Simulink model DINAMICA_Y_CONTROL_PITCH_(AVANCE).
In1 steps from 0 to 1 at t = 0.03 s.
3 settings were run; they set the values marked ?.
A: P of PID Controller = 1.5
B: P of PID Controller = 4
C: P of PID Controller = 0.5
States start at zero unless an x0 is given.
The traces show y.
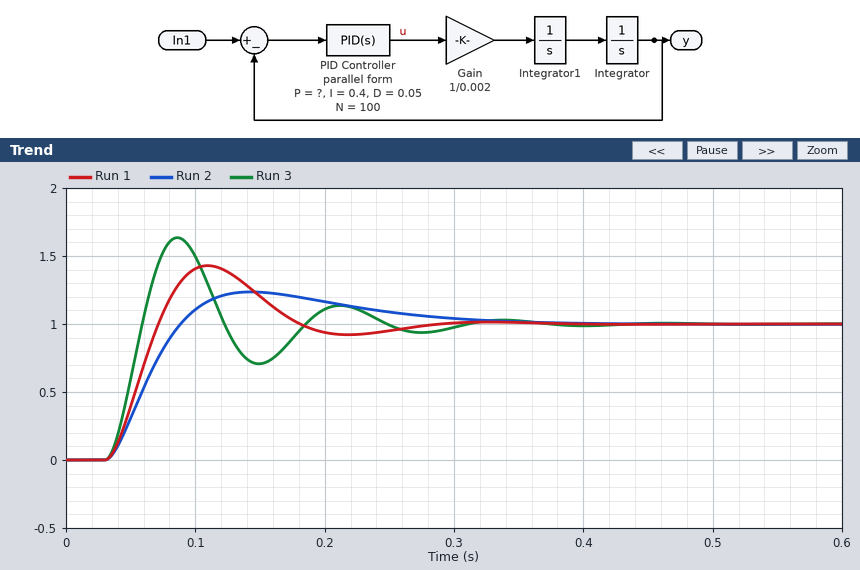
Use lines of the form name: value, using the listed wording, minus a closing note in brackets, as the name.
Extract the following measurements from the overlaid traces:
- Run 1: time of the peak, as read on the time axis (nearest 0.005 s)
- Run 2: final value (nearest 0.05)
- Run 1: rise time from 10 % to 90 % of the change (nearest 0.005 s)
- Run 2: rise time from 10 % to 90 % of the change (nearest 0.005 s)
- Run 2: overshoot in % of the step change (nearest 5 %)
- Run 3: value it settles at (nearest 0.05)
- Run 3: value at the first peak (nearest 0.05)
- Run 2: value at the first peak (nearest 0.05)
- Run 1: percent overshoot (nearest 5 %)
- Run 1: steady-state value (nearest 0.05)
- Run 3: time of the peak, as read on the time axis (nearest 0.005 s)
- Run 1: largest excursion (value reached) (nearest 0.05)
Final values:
Run 1: time of the peak, as read on the time axis: 0.110 s
Run 2: final value: 1.00
Run 1: rise time from 10 % to 90 % of the change: 0.030 s
Run 2: rise time from 10 % to 90 % of the change: 0.040 s
Run 2: overshoot in % of the step change: 25 %
Run 3: value it settles at: 1.00
Run 3: value at the first peak: 1.65
Run 2: value at the first peak: 1.25
Run 1: percent overshoot: 45 %
Run 1: steady-state value: 1.00
Run 3: time of the peak, as read on the time axis: 0.085 s
Run 1: largest excursion (value reached): 1.45
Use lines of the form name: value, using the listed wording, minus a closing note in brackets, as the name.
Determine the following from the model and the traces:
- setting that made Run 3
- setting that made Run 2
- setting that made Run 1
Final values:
setting that made Run 3: B
setting that made Run 2: C
setting that made Run 1: A
